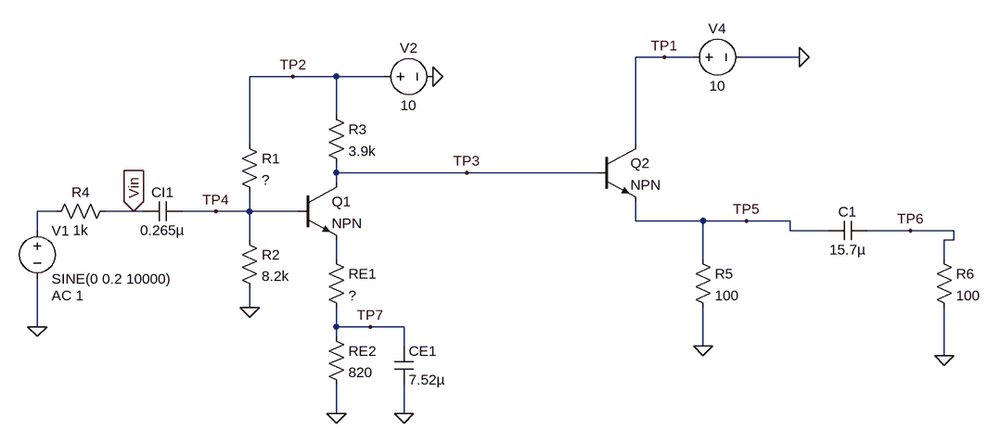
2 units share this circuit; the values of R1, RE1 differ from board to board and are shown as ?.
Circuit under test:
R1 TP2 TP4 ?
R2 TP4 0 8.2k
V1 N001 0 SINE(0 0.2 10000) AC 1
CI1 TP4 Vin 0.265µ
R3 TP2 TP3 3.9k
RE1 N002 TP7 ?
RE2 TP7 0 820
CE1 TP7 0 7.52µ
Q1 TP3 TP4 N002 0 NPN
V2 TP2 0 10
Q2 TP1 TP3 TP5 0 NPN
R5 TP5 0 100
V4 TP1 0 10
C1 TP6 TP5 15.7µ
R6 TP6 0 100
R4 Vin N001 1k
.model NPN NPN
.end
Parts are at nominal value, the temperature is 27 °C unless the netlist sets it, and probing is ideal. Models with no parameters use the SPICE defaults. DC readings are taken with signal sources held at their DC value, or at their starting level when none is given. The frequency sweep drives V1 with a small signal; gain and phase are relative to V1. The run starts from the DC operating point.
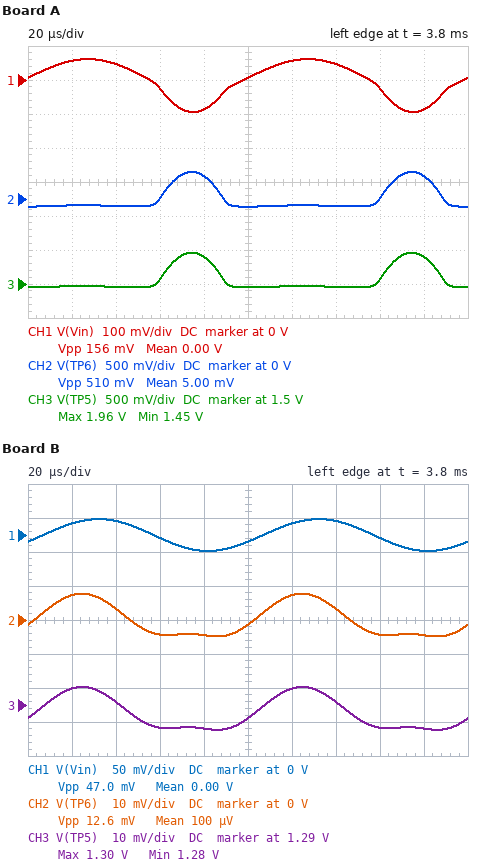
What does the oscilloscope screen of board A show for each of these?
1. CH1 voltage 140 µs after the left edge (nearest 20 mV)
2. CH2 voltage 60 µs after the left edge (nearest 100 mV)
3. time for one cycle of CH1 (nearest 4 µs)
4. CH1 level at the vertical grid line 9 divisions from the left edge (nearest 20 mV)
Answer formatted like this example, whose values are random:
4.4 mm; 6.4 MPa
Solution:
40 mV; 0 V; 100 µs; -80 mV
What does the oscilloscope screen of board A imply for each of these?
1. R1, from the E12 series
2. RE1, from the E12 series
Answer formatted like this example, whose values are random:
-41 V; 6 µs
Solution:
15 kΩ; 330 Ω
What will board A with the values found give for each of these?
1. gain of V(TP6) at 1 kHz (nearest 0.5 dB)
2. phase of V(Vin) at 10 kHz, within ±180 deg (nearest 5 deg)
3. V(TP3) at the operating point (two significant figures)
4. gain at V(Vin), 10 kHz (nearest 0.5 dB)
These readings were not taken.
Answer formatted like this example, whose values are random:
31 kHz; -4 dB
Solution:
-33.0 dB; -10 deg; 2.3 V; -12.0 dB
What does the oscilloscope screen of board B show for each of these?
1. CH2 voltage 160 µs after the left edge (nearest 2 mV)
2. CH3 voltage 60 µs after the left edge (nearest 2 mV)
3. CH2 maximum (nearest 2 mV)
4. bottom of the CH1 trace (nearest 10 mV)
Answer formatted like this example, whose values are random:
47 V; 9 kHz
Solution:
-4 mV; 1.284 V; 8 mV; -20 mV
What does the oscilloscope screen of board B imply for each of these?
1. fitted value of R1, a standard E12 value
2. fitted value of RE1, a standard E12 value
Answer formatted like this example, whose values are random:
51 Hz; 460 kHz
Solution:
10 kΩ; 100 Ω
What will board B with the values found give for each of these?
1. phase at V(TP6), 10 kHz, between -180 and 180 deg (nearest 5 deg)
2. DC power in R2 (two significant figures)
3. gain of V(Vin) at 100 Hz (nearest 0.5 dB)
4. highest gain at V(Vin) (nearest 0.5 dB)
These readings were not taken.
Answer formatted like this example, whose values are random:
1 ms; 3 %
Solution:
0 deg; 1.0 mW; 0 dB; 0 dB
